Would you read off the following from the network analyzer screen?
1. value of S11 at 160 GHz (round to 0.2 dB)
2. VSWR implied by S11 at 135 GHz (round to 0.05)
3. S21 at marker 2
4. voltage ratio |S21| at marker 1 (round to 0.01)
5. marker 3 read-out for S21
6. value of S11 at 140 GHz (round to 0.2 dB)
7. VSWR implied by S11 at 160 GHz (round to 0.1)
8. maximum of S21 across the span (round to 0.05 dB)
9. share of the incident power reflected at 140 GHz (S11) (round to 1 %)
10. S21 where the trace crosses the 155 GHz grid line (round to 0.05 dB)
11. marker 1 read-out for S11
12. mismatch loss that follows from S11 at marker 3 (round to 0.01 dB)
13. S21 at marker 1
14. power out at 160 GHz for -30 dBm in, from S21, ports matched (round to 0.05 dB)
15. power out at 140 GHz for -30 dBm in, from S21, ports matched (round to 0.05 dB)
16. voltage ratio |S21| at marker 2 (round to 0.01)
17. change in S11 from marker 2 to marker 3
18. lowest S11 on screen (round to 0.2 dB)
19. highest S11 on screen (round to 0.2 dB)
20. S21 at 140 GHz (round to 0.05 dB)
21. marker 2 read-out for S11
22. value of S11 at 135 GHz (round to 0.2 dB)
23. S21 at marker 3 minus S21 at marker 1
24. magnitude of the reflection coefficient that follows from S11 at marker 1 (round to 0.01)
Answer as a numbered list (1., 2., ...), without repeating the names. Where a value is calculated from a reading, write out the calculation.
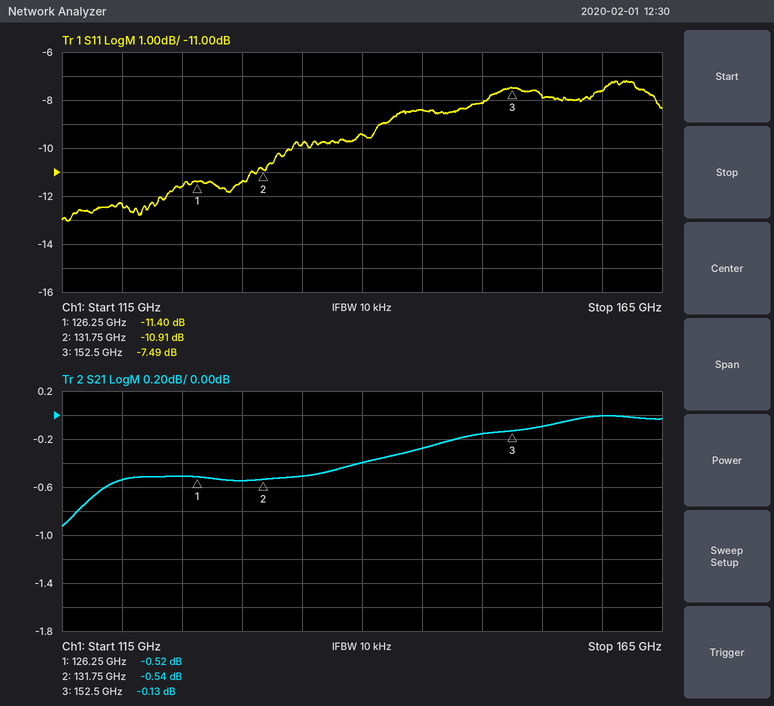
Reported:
1. -7.6 dB
2. |Γ| = 10^(-9.8/20) = 0.3236; VSWR = (1 + 0.3236)/(1 − 0.3236) ≈ 1.96, so 1.95 to the nearest 0.05
3. -0.54 dB
4. 10^(-0.52/20) ≈ 0.94
5. -0.13 dB
6. -9.4 dB
7. |Γ| = 10^(-7.6/20) = 0.4169; VSWR = (1 + 0.4169)/(1 − 0.4169) ≈ 2.4
8. 0.00 dB
9. 10^(-9.4/10) ≈ 11 %
10. -0.10 dB
11. -11.40 dB
12. −10 log10(1 − 10^(-7.49/10)) ≈ 0.85 dB
13. -0.52 dB
14. -30 dBm + (0.00 dB) = -30.00 dBm
15. -30 dBm + (-0.40 dB) = -30.40 dBm
16. 10^(-0.54/20) ≈ 0.94
17. -7.49 − (-10.91) = 3.42 dB
18. -13.0 dB
19. -7.2 dB
20. -0.40 dB
21. -10.91 dB
22. -9.8 dB
23. -0.13 − (-0.52) = 0.39 dB
24. 10^(-11.4/20) ≈ 0.27
